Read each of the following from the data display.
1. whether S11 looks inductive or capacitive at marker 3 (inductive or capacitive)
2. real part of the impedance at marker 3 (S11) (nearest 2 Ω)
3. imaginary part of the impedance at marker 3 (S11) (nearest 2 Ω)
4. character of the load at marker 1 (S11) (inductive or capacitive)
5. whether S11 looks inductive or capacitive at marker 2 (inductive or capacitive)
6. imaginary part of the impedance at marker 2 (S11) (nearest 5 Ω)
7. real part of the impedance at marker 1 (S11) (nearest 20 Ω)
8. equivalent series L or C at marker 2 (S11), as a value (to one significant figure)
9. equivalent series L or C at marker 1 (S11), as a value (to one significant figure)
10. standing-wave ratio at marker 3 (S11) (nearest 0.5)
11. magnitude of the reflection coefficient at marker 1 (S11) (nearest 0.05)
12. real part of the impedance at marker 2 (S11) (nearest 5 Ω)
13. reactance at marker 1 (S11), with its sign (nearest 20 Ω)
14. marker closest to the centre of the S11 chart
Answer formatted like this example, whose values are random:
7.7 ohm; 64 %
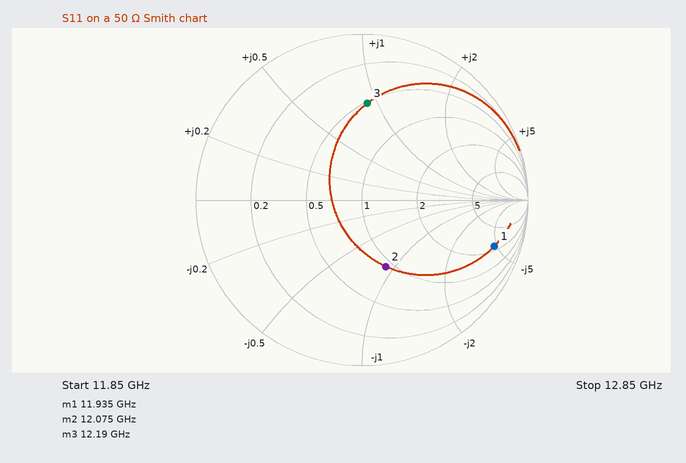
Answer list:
inductive; 26 Ω; +46 Ω; capacitive; capacitive; -45 Ω; 120 Ω; 300 fF; 60 fF; 4.0; 0.85; 45 Ω; -240 Ω; marker 2
